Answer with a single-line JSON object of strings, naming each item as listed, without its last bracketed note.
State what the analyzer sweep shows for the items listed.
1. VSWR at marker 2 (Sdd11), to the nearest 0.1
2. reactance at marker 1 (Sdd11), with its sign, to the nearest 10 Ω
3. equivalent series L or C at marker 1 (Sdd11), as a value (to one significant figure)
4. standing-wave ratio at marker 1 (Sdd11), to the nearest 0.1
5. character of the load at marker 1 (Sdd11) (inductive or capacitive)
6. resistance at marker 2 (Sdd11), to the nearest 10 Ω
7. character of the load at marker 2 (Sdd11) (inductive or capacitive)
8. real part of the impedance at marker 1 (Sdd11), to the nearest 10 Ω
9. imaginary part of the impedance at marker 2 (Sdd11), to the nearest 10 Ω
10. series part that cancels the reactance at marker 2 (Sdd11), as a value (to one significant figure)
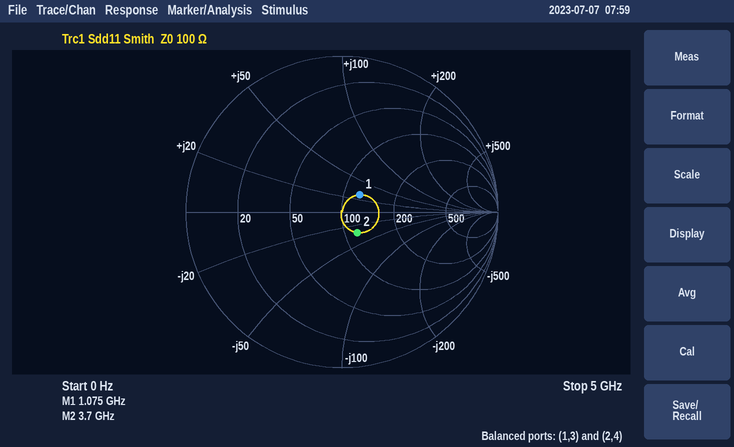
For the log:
{"VSWR at marker 2 (Sdd11), to the nearest 0.1": "1.4", "reactance at marker 1 (Sdd11), with its sign, to the nearest 10 Ω": "+30 Ω", "equivalent series L or C at marker 1 (Sdd11), as a value": "4 nH", "standing-wave ratio at marker 1 (Sdd11), to the nearest 0.1": "1.4", "character of the load at marker 1 (Sdd11)": "inductive", "resistance at marker 2 (Sdd11), to the nearest 10 Ω": "120 Ω", "character of the load at marker 2 (Sdd11)": "capacitive", "real part of the impedance at marker 1 (Sdd11), to the nearest 10 Ω": "120 Ω", "imaginary part of the impedance at marker 2 (Sdd11), to the nearest 10 Ω": "-30 Ω", "series part that cancels the reactance at marker 2 (Sdd11), as a value": "1 nH"}
